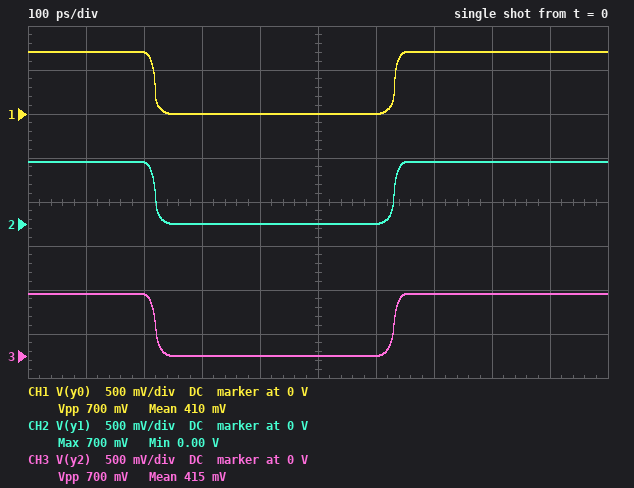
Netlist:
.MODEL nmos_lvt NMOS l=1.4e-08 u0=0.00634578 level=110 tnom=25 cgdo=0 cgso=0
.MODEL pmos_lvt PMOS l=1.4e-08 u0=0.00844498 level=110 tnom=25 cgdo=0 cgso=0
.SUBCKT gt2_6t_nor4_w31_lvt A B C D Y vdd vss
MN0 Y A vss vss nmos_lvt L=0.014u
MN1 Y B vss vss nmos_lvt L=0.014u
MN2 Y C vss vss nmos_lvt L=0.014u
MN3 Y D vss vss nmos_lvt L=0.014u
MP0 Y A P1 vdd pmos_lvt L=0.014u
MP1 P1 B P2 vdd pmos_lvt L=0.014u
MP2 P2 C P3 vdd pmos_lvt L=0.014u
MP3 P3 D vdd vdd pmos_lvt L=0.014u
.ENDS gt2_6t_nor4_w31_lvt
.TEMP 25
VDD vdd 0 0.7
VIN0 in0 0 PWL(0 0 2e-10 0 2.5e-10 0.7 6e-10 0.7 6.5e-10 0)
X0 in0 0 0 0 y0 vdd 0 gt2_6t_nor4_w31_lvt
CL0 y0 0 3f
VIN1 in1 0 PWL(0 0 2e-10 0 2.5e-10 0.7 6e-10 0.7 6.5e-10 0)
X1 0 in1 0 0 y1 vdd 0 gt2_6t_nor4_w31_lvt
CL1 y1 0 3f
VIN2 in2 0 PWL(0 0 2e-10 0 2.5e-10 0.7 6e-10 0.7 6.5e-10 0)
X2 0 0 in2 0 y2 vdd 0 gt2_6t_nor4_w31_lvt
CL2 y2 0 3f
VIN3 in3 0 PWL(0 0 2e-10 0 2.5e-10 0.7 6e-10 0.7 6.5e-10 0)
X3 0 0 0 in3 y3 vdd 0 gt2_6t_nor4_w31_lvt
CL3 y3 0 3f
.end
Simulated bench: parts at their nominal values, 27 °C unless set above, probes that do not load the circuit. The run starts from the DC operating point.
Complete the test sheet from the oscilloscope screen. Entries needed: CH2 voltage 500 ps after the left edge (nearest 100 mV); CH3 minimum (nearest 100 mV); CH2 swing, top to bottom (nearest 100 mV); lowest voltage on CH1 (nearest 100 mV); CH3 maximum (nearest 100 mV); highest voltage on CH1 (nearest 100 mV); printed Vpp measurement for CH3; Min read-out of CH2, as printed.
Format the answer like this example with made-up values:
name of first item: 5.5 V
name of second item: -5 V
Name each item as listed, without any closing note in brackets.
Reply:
CH2 voltage 500 ps after the left edge: 0 V
CH3 minimum: 0 V
CH2 swing, top to bottom: 700 mV
lowest voltage on CH1: 0 V
CH3 maximum: 700 mV
highest voltage on CH1: 700 mV
printed Vpp measurement for CH3: 700 mV
Min read-out of CH2, as printed: 0.00 V
